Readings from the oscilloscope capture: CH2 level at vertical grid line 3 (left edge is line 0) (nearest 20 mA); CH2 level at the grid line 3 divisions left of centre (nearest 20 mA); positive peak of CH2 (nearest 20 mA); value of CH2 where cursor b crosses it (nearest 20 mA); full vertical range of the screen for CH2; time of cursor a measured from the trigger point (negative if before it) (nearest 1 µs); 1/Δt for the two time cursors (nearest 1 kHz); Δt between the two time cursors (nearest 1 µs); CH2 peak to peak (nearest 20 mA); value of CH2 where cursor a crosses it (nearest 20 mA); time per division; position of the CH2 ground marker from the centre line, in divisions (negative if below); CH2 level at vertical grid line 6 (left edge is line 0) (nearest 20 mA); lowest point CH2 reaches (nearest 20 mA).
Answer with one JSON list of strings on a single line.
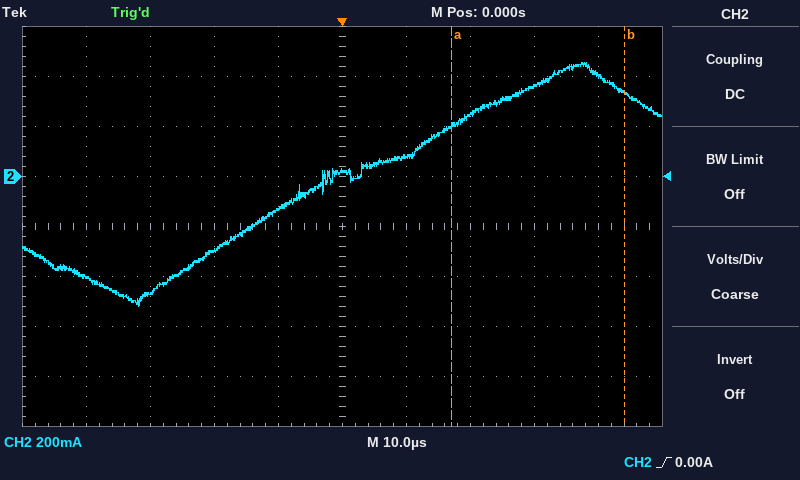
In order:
["-300 mA", "-460 mA", "460 mA", "340 mA", "1.6 A", "+17 µs", "37 kHz", "27 µs", "980 mA", "200 mA", "10 µs", "+1.0 div", "80 mA", "-520 mA"]
